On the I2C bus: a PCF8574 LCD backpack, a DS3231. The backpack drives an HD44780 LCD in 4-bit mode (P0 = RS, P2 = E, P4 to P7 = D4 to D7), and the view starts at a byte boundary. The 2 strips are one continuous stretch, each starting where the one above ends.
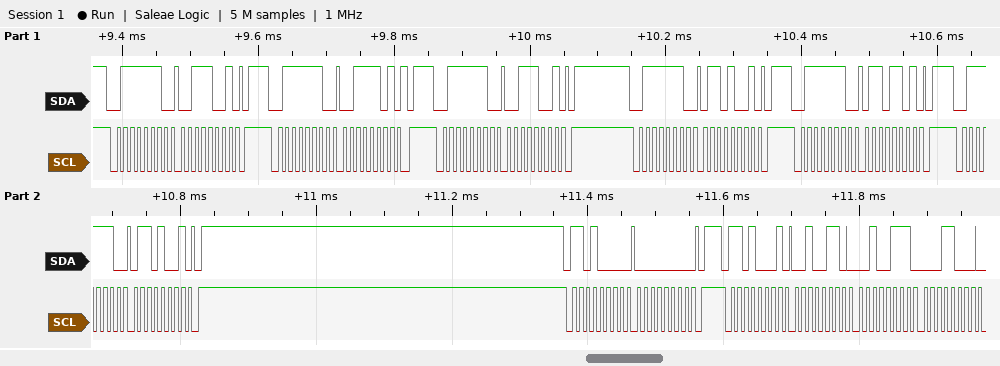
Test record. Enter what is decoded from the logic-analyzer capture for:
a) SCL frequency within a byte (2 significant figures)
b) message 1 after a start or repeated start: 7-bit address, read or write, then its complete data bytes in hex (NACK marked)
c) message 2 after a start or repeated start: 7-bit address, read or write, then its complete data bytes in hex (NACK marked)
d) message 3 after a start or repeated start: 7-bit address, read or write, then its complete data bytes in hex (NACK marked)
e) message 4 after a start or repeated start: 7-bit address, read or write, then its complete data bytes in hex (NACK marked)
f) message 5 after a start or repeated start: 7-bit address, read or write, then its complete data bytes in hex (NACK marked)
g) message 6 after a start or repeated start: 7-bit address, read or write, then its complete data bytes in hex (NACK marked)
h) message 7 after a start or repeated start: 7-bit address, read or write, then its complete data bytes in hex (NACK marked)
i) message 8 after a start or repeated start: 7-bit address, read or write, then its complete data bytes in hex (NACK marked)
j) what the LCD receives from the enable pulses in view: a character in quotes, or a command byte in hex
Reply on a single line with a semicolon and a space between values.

100 kHz; 0x3F write: 39; 0x3F write: 3D; 0x3F write: 39; 0x3F write: 69; 0x3F write: 6D; 0x3F write: 69; 0x68 write: 00; 0x68 read: 26 27 18; '6'
